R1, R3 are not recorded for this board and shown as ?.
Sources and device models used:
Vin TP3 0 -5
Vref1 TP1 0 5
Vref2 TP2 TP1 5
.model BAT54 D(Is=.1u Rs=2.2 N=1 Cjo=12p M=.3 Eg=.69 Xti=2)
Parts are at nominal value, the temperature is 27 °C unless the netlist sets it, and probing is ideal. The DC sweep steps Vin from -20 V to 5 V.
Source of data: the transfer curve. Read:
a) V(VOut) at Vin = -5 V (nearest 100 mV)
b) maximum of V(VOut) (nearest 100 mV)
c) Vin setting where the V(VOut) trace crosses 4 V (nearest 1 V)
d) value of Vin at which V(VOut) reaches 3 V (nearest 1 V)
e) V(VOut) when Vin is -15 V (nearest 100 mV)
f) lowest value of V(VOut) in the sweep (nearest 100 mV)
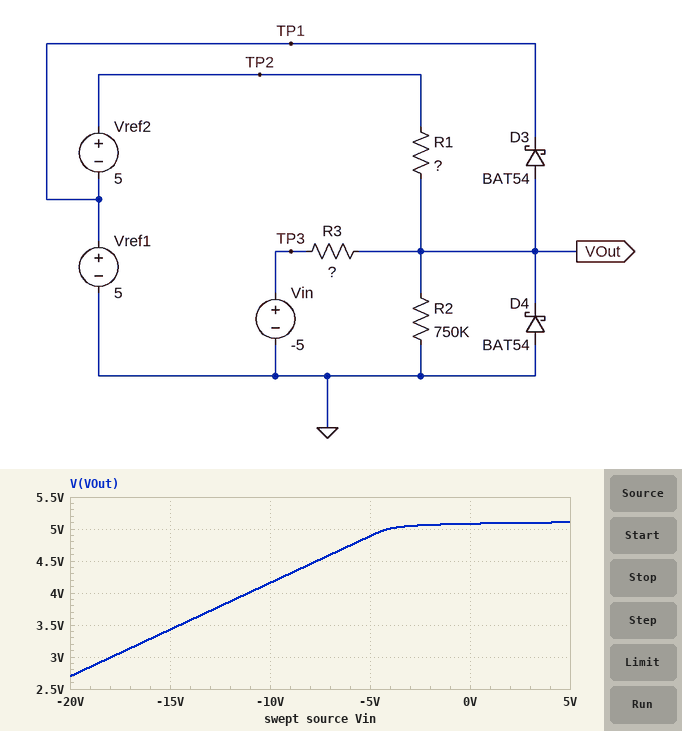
4.9 V
5.1 V
-11 V
-18 V
3.4 V
2.7 V
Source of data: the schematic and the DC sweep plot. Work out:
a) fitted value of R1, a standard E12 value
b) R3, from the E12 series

390 kΩ
1.5 MΩ
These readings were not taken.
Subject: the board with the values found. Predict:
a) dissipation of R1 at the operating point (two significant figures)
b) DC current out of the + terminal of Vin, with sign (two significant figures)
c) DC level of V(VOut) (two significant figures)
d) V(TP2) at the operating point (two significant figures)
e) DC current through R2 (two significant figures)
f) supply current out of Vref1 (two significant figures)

67 µW
-6.6 µA
4.9 V
10 V
6.5 µA
13 µA
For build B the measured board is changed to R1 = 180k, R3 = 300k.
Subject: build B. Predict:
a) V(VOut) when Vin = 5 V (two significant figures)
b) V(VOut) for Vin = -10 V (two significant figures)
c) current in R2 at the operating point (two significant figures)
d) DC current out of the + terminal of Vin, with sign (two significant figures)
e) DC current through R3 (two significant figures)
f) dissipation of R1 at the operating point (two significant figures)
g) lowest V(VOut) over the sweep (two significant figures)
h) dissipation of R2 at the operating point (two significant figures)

5.1 V
2.2 V
5.1 µA
-29 µA
29 µA
210 µW
-120 mV
19 µW
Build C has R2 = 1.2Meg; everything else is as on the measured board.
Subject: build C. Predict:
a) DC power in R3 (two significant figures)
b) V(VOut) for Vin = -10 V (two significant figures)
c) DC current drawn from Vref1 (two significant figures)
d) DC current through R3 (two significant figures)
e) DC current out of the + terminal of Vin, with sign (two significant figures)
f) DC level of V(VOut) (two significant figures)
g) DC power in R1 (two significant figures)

68 µW
4.7 V
11 µA
6.7 µA
-6.7 µA
5.1 V
62 µW
